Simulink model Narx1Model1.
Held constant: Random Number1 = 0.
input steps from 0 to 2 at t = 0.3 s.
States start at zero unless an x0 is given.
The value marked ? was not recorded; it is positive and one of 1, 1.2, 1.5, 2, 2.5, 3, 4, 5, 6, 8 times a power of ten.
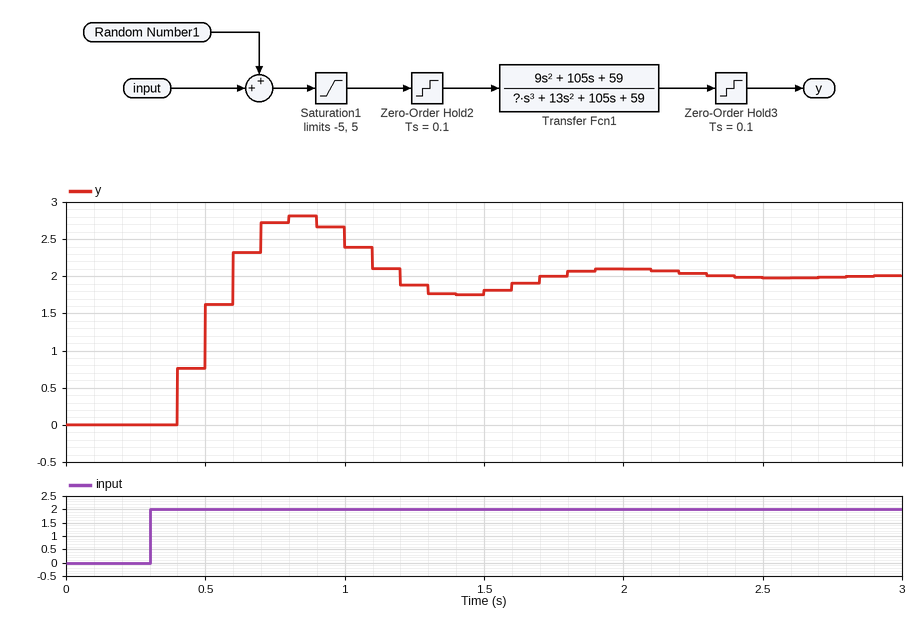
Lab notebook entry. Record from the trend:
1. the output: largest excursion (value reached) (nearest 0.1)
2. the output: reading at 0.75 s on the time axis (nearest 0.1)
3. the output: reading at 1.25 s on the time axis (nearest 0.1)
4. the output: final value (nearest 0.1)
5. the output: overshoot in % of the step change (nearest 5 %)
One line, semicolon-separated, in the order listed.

2.8; 2.7; 1.9; 2.0; 40 %
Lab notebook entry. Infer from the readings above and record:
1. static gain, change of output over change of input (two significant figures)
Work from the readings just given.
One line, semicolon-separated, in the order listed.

1.0
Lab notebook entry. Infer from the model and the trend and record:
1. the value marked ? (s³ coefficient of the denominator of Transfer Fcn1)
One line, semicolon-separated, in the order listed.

3
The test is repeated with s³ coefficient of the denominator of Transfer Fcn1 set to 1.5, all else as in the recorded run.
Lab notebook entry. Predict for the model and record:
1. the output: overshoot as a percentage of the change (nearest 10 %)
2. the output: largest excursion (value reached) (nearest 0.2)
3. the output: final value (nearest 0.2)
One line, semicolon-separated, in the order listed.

20 %; 2.4; 2.0
